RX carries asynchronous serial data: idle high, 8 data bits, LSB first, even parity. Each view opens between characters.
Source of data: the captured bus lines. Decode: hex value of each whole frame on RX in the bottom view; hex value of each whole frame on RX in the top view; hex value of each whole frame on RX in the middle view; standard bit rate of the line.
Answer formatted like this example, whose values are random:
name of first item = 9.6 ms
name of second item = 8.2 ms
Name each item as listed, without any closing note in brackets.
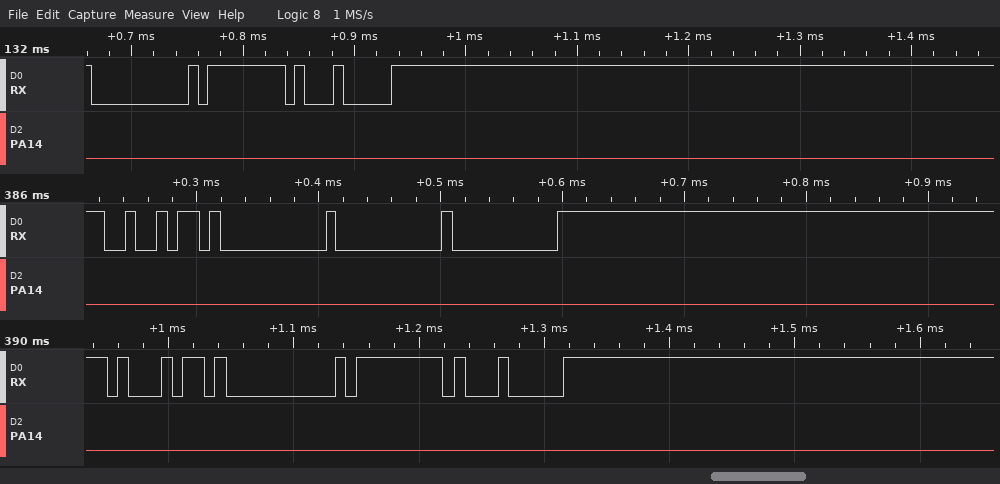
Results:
hex value of each whole frame on RX in the bottom view = D1, 00, FF, 04
hex value of each whole frame on RX in the top view = 00, FF, 04
hex value of each whole frame on RX in the middle view = D2, 00, 00, 00
standard bit rate of the line = 115200 baud
